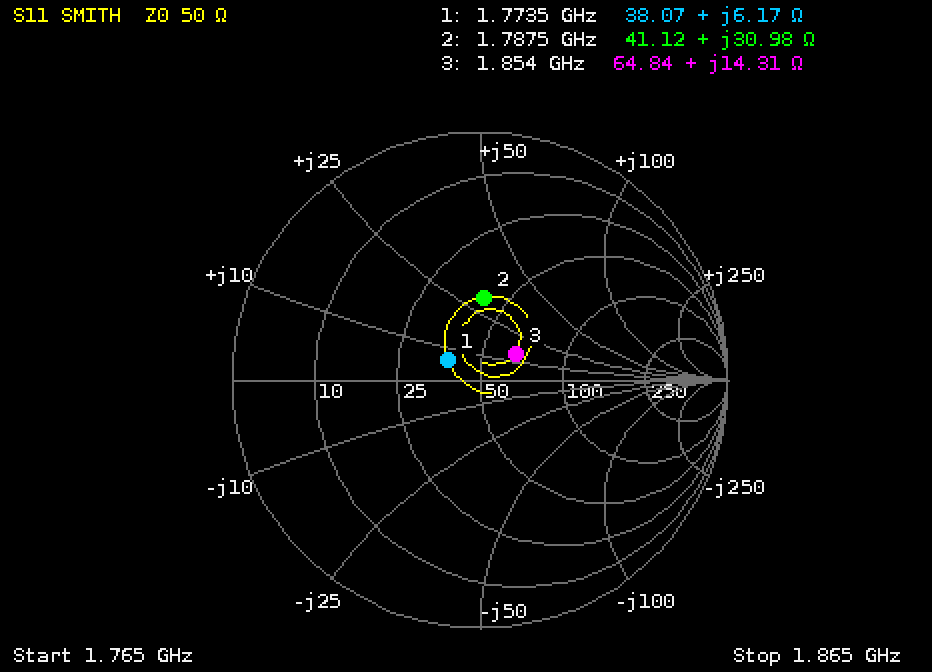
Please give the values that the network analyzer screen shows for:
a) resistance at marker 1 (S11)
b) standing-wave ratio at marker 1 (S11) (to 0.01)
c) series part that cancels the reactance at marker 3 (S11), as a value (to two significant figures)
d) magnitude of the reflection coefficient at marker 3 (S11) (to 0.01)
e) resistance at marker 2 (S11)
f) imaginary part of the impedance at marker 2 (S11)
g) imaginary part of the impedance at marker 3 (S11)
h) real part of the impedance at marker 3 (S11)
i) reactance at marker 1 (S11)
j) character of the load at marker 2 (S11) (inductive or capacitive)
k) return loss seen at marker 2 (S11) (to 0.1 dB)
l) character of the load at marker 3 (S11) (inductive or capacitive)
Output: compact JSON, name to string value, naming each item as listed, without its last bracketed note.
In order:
{"resistance at marker 1": "38.07 Ω", "standing-wave ratio at marker 1 (S11)": "1.36", "series part that cancels the reactance at marker 3 (S11), as a value": "6.0 pF", "magnitude of the reflection coefficient at marker 3 (S11)": "0.18", "resistance at marker 2": "41.12 Ω", "imaginary part of the impedance at marker 2": "+30.98 Ω", "imaginary part of the impedance at marker 3": "+14.31 Ω", "real part of the impedance at marker 3": "64.84 Ω", "reactance at marker 1": "+6.17 Ω", "character of the load at marker 2 (S11)": "inductive", "return loss seen at marker 2 (S11)": "9.5 dB", "character of the load at marker 3 (S11)": "inductive"}
